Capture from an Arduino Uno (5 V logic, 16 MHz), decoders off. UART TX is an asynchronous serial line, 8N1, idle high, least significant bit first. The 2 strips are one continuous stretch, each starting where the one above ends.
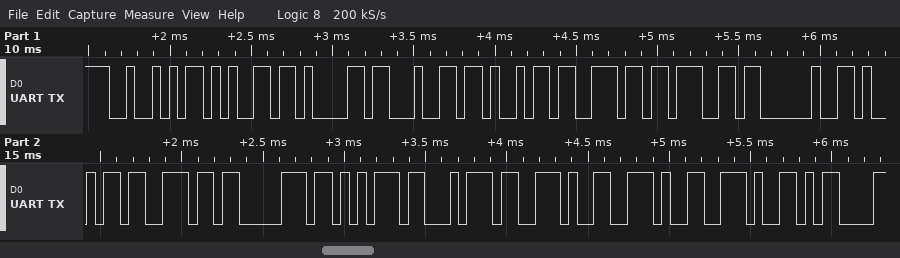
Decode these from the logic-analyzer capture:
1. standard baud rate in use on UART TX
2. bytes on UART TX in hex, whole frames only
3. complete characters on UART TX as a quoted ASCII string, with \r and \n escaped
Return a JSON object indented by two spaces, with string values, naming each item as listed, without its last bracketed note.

{
  "standard baud rate in use on UART TX": "19200 baud",
  "bytes on UART TX in hex, whole frames only": "52 65 61 64 69 6E 67 20 69 6E 70 75 74 2E 2E 2E 0D",
  "complete characters on UART TX as a quoted ASCII string, with \\r and \\n escaped": "\"Reading input...\\r\""
}
